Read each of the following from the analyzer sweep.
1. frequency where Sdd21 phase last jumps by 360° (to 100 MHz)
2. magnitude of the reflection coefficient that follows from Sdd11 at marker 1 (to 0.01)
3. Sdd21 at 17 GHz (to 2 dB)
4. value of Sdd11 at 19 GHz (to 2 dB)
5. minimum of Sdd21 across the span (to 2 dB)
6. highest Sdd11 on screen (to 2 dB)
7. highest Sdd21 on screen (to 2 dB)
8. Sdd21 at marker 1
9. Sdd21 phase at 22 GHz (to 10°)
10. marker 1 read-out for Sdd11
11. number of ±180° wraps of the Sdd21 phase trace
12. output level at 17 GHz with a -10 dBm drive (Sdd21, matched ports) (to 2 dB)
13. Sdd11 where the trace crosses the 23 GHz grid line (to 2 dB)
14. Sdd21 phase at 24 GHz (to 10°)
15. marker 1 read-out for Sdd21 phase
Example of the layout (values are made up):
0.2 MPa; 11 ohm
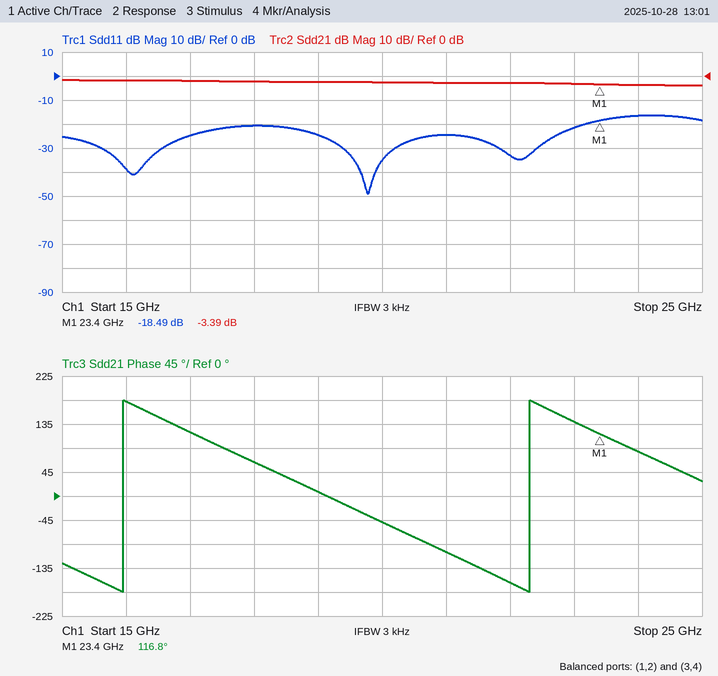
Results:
22.3 GHz; 0.12; -2 dB; -24 dB; -4 dB; -16 dB; -2 dB; -3.39 dB; -160°; -18.49 dB; 2; -12 dBm; -22 dB; 80°; 116.8°
